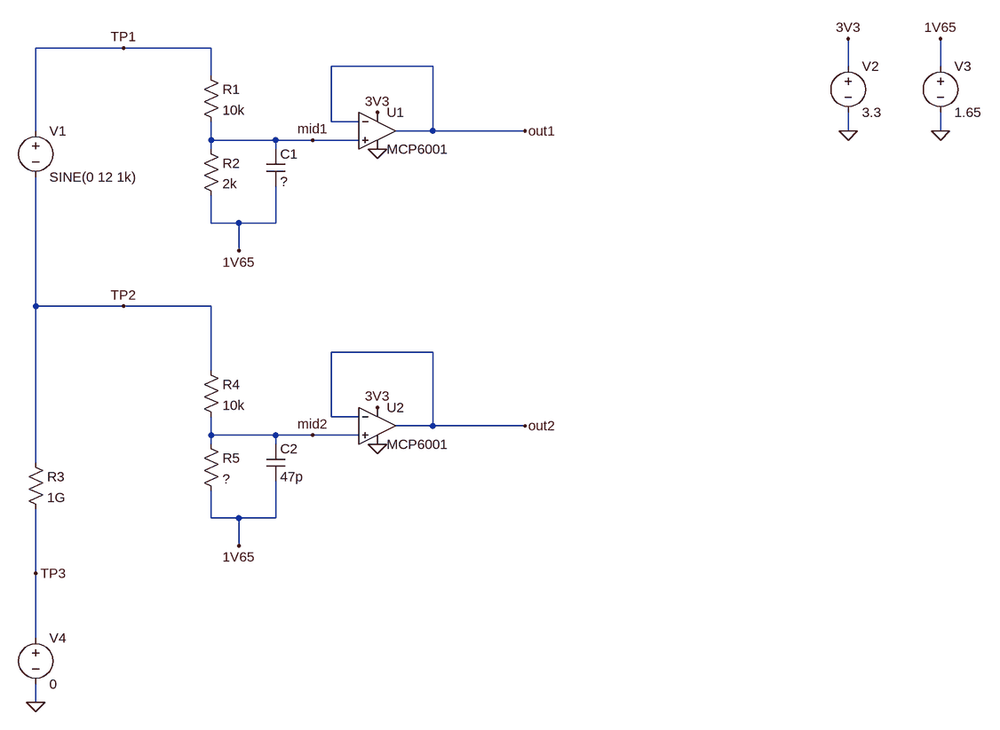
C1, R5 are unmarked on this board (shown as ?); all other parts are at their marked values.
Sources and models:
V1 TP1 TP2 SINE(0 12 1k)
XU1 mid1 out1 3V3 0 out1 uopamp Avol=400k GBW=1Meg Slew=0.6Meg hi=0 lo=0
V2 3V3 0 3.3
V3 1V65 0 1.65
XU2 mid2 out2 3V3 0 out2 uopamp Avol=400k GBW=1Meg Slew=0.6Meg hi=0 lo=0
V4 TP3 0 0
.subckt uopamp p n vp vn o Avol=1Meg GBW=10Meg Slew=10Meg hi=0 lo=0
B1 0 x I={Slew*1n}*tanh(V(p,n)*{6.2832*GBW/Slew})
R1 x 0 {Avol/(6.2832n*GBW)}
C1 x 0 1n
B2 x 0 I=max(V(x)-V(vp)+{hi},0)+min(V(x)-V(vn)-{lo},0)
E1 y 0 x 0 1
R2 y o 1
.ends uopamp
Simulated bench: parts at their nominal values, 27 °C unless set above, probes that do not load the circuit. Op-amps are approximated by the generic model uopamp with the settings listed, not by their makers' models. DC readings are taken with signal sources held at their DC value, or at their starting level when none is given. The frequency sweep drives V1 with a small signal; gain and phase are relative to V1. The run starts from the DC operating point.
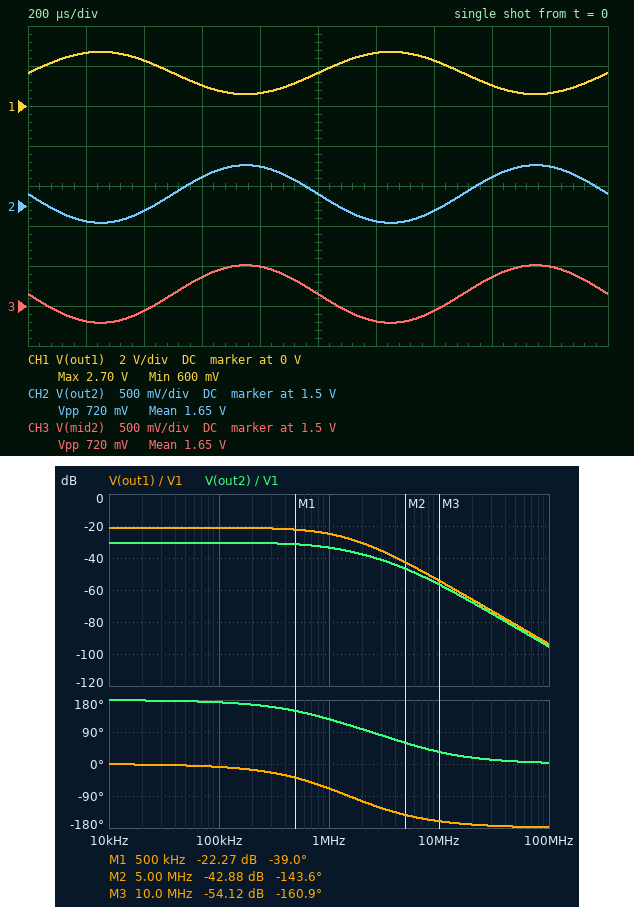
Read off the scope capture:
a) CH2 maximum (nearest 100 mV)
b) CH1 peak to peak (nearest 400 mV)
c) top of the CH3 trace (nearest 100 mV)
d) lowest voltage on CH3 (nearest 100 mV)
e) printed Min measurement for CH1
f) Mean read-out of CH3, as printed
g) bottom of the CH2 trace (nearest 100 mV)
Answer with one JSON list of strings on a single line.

["2.0 V", "2.0 V", "2.0 V", "1.3 V", "600 mV", "1.65 V", "1.3 V"]
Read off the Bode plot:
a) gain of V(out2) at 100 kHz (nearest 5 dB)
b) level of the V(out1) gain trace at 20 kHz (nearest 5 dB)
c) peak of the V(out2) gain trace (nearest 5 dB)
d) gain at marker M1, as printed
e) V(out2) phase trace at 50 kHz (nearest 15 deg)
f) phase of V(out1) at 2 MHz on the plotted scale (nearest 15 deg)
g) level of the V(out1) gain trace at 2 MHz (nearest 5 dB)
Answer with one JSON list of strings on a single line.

["-30 dB", "-20 dB", "-30 dB", "-22.27 dB", "180 deg", "-105 deg", "-30 dB"]
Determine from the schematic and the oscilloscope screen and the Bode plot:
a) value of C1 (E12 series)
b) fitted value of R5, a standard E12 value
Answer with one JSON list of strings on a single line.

["39 pF", "680 Ω"]
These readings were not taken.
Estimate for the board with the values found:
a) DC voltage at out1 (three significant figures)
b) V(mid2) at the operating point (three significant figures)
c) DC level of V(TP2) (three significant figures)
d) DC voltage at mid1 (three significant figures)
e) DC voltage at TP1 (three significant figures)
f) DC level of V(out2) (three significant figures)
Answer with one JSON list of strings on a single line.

["1.65 V", "1.65 V", "1.65 V", "1.65 V", "1.65 V", "1.65 V"]
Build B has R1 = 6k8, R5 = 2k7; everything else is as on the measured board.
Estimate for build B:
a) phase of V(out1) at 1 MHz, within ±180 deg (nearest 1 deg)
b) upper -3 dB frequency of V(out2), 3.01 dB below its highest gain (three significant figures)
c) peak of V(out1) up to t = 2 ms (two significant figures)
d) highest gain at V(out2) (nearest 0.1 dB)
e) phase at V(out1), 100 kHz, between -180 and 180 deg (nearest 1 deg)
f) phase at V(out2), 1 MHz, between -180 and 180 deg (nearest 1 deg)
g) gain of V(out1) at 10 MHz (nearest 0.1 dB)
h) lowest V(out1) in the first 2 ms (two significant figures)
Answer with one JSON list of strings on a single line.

["-65 deg", "766 kHz", "2.8 V", "-18.0 dB", "-8 deg", "102 deg", "-52.6 dB", "530 mV"]
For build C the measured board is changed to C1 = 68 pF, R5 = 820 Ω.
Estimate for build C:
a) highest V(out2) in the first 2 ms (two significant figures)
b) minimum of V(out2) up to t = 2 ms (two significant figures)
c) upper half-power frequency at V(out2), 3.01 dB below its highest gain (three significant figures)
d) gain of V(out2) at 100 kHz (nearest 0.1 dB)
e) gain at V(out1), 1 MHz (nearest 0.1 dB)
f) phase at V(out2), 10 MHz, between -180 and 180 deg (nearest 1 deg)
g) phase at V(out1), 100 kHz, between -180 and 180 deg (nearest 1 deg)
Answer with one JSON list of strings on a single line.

["2.1 V", "1.2 V", "1.02 MHz", "-28.9 dB", "-26.2 dB", "30 deg", "-10 deg"]
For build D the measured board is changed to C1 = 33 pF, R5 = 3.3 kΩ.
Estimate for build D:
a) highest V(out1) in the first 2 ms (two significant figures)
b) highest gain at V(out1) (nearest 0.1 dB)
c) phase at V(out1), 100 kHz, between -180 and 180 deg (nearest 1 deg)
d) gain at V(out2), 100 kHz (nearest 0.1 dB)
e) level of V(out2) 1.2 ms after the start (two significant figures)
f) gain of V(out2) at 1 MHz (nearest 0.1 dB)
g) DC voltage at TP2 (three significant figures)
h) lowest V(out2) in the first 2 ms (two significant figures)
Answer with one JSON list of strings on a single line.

["2.6 V", "-22.0 dB", "-7 deg", "-17.8 dB", "160 mV", "-23.0 dB", "1.65 V", "85 mV"]
